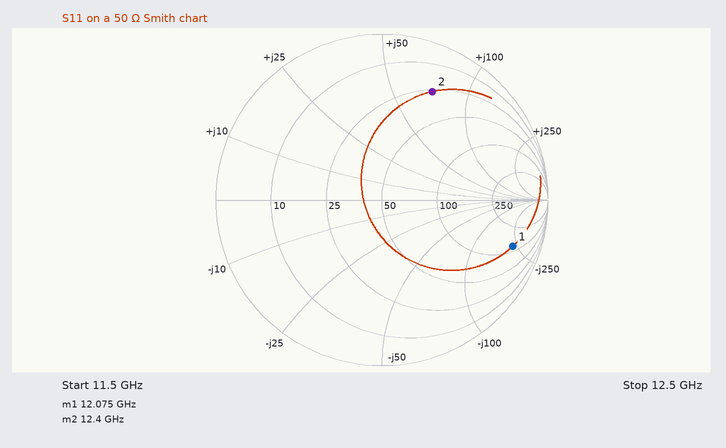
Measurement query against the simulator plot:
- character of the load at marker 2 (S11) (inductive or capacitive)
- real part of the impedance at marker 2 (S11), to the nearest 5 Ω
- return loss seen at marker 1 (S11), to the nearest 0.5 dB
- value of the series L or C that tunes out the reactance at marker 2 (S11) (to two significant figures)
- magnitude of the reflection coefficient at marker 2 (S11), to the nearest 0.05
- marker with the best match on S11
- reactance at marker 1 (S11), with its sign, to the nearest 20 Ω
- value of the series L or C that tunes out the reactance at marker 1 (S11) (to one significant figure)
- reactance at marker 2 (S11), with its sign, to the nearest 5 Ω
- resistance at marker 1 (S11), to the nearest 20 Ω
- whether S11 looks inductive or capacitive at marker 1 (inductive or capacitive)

inductive
25 Ω
1.5 dB
180 fF
0.70
marker 2
-220 Ω
3 nH
+70 Ω
120 Ω
capacitive
